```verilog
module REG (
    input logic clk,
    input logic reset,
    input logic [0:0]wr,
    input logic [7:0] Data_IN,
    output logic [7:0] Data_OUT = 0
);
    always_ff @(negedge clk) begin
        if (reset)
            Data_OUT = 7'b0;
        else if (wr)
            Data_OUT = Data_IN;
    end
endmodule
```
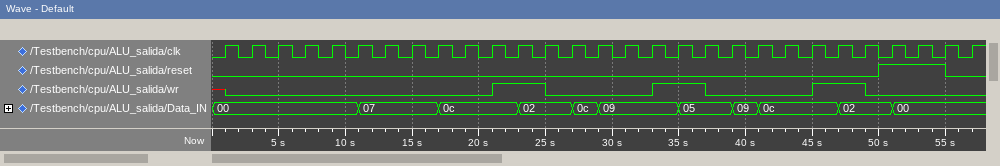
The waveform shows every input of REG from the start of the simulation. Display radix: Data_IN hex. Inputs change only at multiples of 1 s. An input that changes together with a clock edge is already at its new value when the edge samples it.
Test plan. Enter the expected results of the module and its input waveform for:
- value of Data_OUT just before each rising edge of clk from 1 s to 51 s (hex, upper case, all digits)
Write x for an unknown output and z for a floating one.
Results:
00, 00, 00, 00, 00, 00, 00, 00, 00, 00, 00, 0C, 02, 02, 02, 02, 02, 09, 05, 05, 05, 05, 05, 0C, 02, 00
